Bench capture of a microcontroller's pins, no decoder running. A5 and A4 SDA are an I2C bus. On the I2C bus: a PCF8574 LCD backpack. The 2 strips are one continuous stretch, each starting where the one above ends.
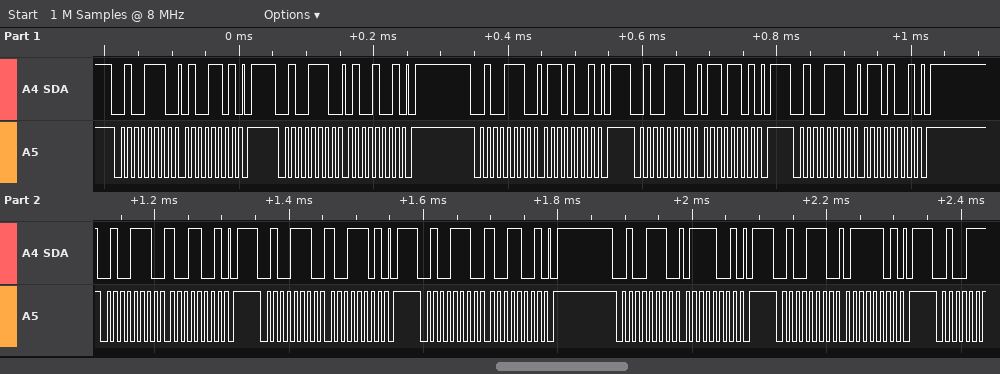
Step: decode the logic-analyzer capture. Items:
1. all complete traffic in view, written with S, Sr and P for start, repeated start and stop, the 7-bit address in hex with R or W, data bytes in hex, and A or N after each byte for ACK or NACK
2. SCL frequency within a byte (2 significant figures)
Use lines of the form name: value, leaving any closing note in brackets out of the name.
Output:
all complete traffic in view, written with S, Sr and P for start, repeated start and stop, the 7-bit address in hex with R or W, data bytes in hex, and A or N after each byte for ACK or NACK: S 27W A 4D A P S 27W A 49 A P S 27W A 69 A P S 27W A 6D A P S 27W A 69 A P S 27W A 99 A P S 27W A 9D A P S 27W A 99 A P S 27W A 79 A P S 27W A 7D A P
SCL frequency within a byte: 100 kHz
